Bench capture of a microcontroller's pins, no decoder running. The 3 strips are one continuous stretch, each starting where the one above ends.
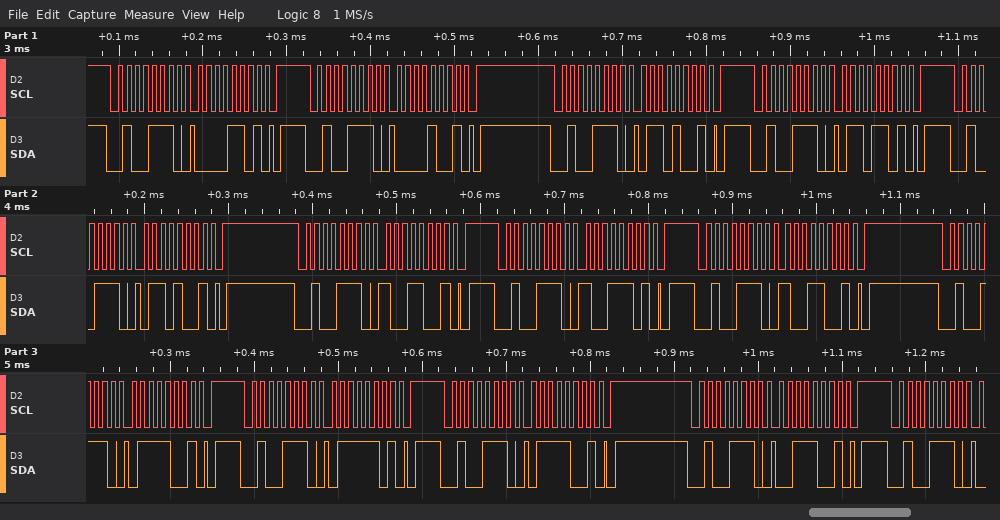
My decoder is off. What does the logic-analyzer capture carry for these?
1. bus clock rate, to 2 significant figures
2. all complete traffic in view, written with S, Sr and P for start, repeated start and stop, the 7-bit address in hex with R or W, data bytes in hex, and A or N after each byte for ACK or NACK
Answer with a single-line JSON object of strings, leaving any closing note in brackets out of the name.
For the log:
{"bus clock rate, to 2 significant figures": "100 kHz", "all complete traffic in view, written with S, Sr and P for start, repeated start and stop, the 7-bit address in hex with R or W, data bytes in hex, and A or N after each byte for ACK or NACK": "S 27W A 0D A P S 27W A 09 A P S 27W A 69 A P S 27W A 6D A P S 27W A 69 A P S 27W A 99 A P S 27W A 9D A P S 27W A 99 A P S 27W A 79 A P S 27W A 7D A P S 27W A 79 A P S 27W A 39 A P S 27W A"}
